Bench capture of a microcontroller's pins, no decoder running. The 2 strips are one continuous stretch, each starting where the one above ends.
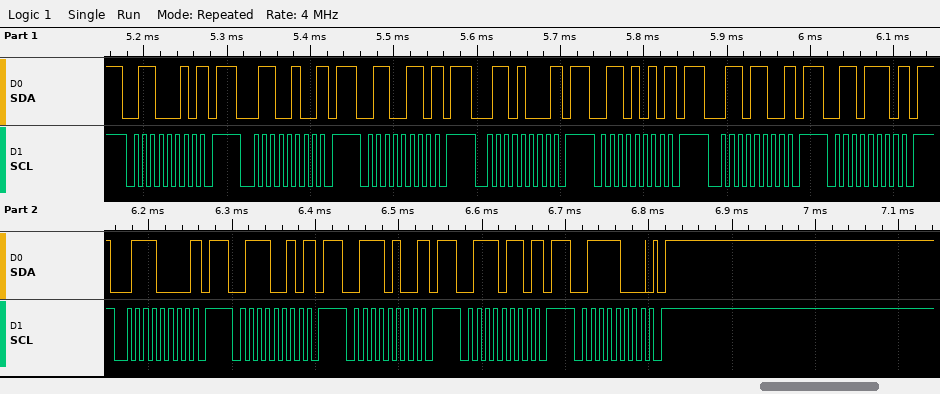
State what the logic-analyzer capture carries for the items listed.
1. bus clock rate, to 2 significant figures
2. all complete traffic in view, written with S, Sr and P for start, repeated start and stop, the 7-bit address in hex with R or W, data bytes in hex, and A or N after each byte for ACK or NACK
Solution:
100 kHz
S 31W N P S 32W N P S 33W N P S 34W N P S 35W N P S 36W N P S 37W N P S 38W N P S 39W N P S 3AW N P S 3BW N P S 3CW A P
